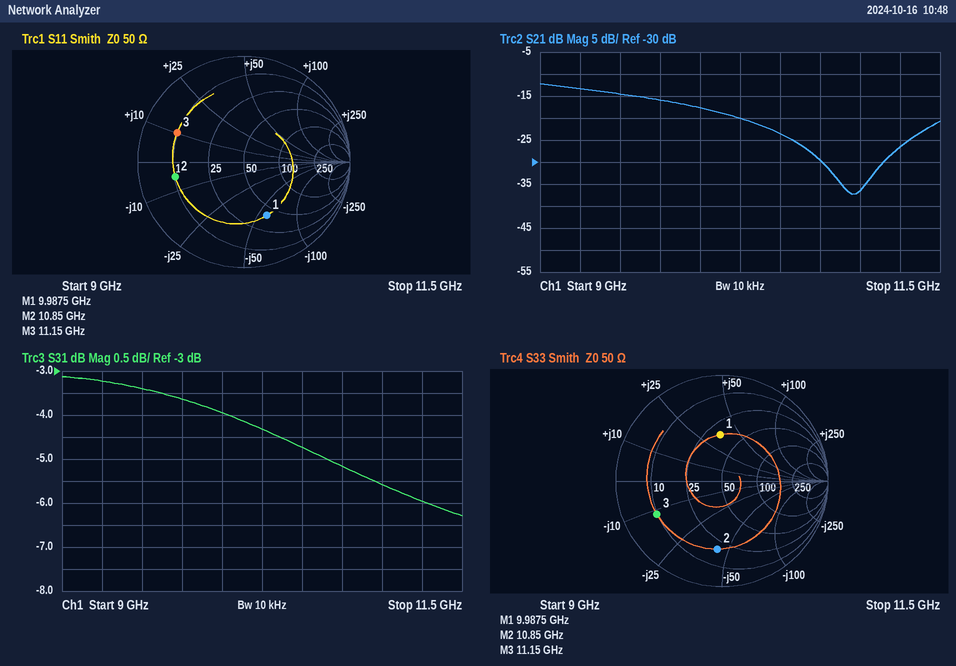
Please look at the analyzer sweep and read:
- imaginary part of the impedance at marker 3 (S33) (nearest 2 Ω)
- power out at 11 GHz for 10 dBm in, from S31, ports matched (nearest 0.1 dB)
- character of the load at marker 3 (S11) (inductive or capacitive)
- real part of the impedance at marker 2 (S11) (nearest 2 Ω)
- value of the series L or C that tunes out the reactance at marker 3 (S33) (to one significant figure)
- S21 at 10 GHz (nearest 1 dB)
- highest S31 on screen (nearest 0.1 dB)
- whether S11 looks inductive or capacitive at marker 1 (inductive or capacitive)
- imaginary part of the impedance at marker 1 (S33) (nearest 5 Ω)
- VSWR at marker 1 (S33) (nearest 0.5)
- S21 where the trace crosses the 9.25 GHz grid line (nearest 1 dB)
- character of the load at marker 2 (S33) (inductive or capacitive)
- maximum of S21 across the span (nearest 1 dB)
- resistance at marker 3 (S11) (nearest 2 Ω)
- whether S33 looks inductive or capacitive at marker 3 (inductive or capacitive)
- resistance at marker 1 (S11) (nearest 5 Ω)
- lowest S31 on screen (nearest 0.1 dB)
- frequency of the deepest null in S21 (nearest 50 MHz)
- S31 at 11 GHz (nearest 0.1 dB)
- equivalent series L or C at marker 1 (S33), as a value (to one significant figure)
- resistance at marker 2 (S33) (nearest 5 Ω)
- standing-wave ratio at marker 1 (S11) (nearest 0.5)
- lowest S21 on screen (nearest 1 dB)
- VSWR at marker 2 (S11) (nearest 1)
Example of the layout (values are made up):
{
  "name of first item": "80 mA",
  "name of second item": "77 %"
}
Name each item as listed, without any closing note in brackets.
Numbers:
{
  "imaginary part of the impedance at marker 3 (S33)": "-12 Ω",
  "power out at 11 GHz for 10 dBm in, from S31, ports matched": "4.4 dBm",
  "character of the load at marker 3 (S11)": "inductive",
  "real part of the impedance at marker 2 (S11)": "10 Ω",
  "value of the series L or C that tunes out the reactance at marker 3 (S33)": "200 pH",
  "S21 at 10 GHz": "-18 dB",
  "highest S31 on screen": "-3.1 dB",
  "whether S11 looks inductive or capacitive at marker 1": "capacitive",
  "imaginary part of the impedance at marker 1 (S33)": "+35 Ω",
  "VSWR at marker 1 (S33)": "2.5",
  "S21 where the trace crosses the 9.25 GHz grid line": "-13 dB",
  "character of the load at marker 2 (S33)": "capacitive",
  "maximum of S21 across the span": "-12 dB",
  "resistance at marker 3 (S11)": "10 Ω",
  "whether S33 looks inductive or capacitive at marker 3": "capacitive",
  "resistance at marker 1 (S11)": "40 Ω",
  "lowest S31 on screen": "-6.3 dB",
  "frequency of the deepest null in S21": "10.95 GHz",
  "S31 at 11 GHz": "-5.6 dB",
  "equivalent series L or C at marker 1 (S33), as a value": "600 pH",
  "resistance at marker 2 (S33)": "20 Ω",
  "standing-wave ratio at marker 1 (S11)": "3.5",
  "lowest S21 on screen": "-37 dB",
  "VSWR at marker 2 (S11)": "5"
}
